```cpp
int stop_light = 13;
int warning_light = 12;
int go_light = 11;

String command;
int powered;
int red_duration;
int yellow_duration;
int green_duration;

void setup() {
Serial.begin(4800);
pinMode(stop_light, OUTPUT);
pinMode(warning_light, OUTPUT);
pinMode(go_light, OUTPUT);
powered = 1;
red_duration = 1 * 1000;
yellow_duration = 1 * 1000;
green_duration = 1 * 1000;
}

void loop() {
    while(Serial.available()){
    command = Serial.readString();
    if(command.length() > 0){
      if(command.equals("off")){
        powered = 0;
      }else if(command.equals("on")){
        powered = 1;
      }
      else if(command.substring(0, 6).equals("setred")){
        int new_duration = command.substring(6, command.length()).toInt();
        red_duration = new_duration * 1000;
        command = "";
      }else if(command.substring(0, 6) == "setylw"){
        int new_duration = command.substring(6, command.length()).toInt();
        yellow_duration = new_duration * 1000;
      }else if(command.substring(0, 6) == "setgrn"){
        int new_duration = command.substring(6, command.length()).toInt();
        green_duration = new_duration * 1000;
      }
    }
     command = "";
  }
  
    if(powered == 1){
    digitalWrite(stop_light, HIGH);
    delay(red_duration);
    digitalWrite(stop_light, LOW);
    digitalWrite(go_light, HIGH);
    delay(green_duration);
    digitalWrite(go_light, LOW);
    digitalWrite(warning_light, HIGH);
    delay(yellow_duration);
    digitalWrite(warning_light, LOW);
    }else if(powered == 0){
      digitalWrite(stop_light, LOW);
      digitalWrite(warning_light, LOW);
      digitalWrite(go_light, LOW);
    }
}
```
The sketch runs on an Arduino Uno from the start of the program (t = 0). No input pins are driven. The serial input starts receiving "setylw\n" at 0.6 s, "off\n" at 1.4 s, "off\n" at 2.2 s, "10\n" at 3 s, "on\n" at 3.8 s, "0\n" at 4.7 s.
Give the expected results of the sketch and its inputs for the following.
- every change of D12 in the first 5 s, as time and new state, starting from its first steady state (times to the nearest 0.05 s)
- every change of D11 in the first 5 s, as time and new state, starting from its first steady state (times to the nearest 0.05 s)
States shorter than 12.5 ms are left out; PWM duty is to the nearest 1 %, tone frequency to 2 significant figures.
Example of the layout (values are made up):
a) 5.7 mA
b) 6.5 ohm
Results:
a) 0 s low; 2 s high; 3 s low
b) 0 s low; 1 s high; 2 s low
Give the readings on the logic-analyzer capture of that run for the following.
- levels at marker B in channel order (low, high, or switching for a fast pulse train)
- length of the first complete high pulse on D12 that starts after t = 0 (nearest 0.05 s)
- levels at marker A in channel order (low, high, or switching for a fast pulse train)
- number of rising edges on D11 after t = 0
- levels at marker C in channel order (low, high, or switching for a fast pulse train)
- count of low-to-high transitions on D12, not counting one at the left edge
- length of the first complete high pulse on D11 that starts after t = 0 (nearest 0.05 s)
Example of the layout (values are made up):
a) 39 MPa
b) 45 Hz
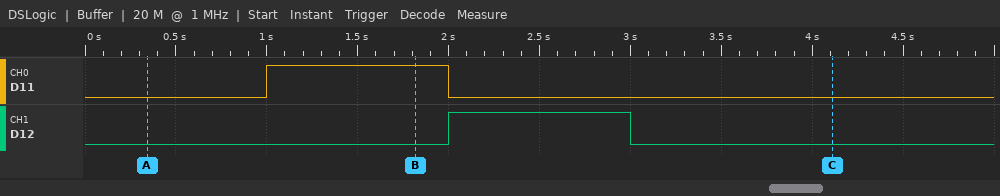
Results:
a) D11 high, D12 low
b) 1.00 s
c) D11 low, D12 low
d) 1
e) D11 low, D12 low
f) 1
g) 1.00 s
